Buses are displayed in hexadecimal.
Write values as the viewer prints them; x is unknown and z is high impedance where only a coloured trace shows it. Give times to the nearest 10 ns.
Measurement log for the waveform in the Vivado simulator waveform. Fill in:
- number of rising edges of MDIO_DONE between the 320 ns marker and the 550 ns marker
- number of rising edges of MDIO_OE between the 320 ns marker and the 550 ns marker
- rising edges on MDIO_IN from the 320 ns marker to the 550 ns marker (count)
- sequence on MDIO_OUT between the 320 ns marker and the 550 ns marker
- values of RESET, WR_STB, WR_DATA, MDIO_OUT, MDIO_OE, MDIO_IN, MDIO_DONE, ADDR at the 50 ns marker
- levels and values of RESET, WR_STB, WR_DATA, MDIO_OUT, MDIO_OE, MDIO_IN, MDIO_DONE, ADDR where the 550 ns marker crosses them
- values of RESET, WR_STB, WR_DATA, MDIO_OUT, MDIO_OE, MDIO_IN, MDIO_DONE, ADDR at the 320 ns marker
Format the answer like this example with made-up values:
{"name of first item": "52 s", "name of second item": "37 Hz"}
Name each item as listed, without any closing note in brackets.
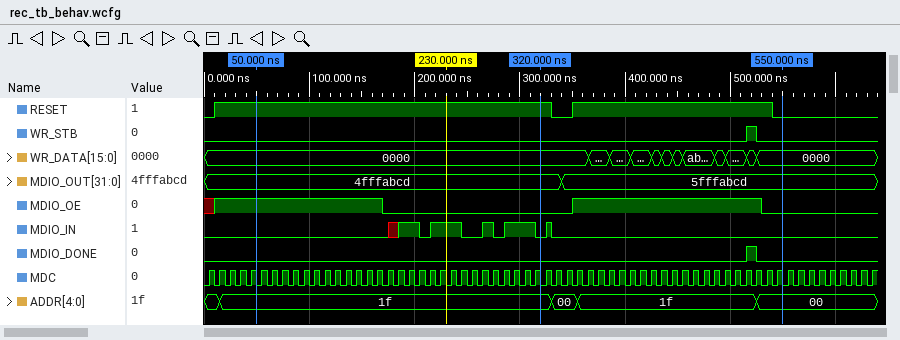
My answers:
{"number of rising edges of MDIO_DONE between the 320 ns marker and the 550 ns marker": "1", "number of rising edges of MDIO_OE between the 320 ns marker and the 550 ns marker": "1", "rising edges on MDIO_IN from the 320 ns marker to the 550 ns marker": "1", "sequence on MDIO_OUT between the 320 ns marker and the 550 ns marker": "4fffabcd, 5fffabcd", "values of RESET, WR_STB, WR_DATA, MDIO_OUT, MDIO_OE, MDIO_IN, MDIO_DONE, ADDR at the 50 ns marker": "RESET=1, WR_STB=0, WR_DATA=0000, MDIO_OUT=4fffabcd, MDIO_OE=1, MDIO_IN=0, MDIO_DONE=0, ADDR=1f", "levels and values of RESET, WR_STB, WR_DATA, MDIO_OUT, MDIO_OE, MDIO_IN, MDIO_DONE, ADDR where the 550 ns marker crosses them": "RESET=0, WR_STB=0, WR_DATA=0000, MDIO_OUT=5fffabcd, MDIO_OE=0, MDIO_IN=0, MDIO_DONE=0, ADDR=00", "values of RESET, WR_STB, WR_DATA, MDIO_OUT, MDIO_OE, MDIO_IN, MDIO_DONE, ADDR at the 320 ns marker": "RESET=1, WR_STB=0, WR_DATA=0000, MDIO_OUT=4fffabcd, MDIO_OE=0, MDIO_IN=0, MDIO_DONE=0, ADDR=1f"}
